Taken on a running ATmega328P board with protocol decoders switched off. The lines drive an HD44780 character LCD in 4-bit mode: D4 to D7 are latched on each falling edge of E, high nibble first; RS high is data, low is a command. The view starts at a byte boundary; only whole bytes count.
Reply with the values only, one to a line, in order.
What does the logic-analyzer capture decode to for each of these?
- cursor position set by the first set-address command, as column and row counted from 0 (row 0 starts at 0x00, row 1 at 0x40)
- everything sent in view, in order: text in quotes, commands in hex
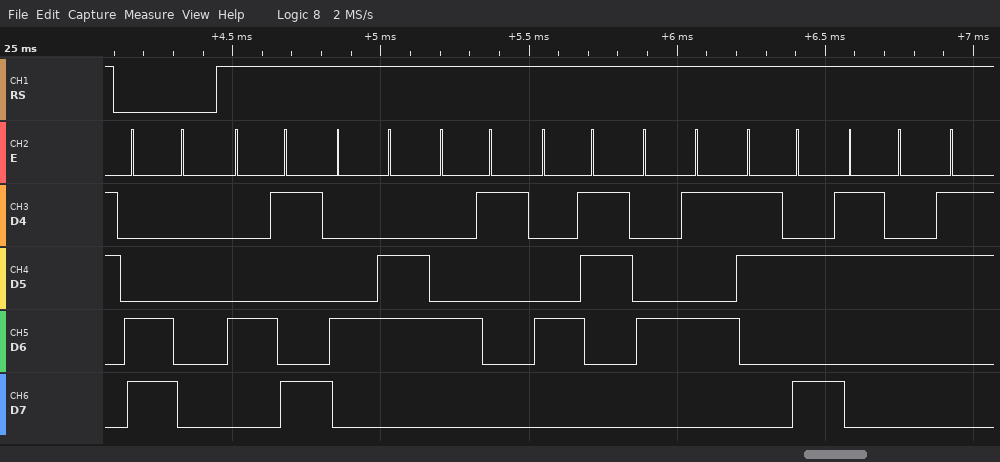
column 0, row 1
0xC0 "IFACE:2"
